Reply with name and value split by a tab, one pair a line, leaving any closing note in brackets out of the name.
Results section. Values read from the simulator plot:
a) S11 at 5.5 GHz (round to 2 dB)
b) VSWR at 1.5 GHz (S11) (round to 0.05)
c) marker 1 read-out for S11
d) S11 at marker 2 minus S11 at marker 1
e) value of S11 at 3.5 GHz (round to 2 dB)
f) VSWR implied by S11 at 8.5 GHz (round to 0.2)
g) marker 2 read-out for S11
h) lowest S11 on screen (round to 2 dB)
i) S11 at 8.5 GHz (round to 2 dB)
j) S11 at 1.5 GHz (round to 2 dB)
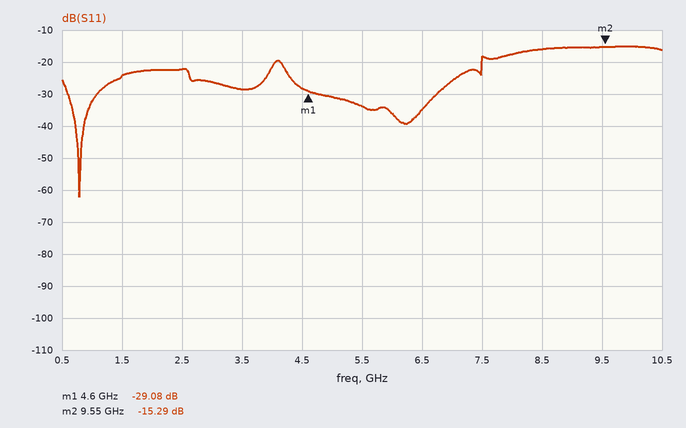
S11 at 5.5 GHz	-34 dB
VSWR at 1.5 GHz (S11)	1.15
marker 1 read-out for S11	-29.08 dB
S11 at marker 2 minus S11 at marker 1	13.79 dB
value of S11 at 3.5 GHz	-28 dB
VSWR implied by S11 at 8.5 GHz	1.4
marker 2 read-out for S11	-15.29 dB
lowest S11 on screen	-62 dB
S11 at 8.5 GHz	-16 dB
S11 at 1.5 GHz	-24 dB
